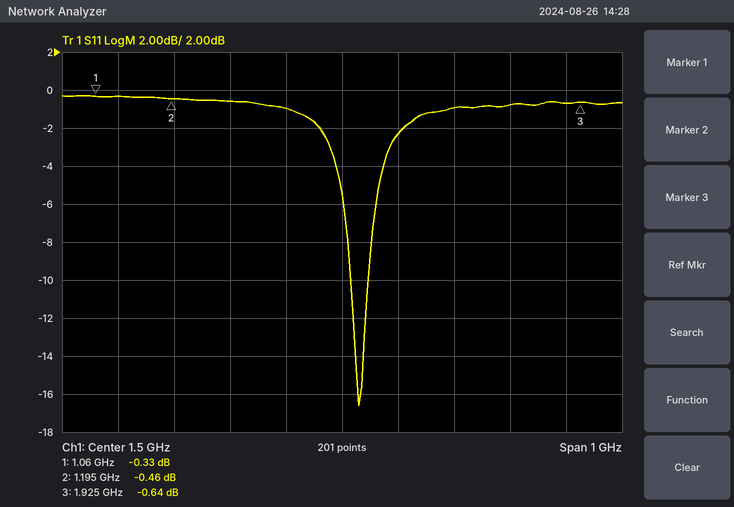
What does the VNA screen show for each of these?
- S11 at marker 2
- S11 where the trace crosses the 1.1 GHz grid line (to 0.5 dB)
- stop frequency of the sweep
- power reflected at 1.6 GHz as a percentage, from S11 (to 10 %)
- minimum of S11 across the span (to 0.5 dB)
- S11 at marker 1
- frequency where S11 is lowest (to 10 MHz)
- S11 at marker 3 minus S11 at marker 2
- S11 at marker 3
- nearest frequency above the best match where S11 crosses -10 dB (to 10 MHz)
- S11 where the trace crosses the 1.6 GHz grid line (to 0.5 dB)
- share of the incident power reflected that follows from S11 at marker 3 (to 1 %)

-0.46 dB
-0.5 dB
2 GHz
60 %
-16.5 dB
-0.33 dB
1.53 GHz
-0.18 dB
-0.64 dB
1.55 GHz
-2.5 dB
86 %
